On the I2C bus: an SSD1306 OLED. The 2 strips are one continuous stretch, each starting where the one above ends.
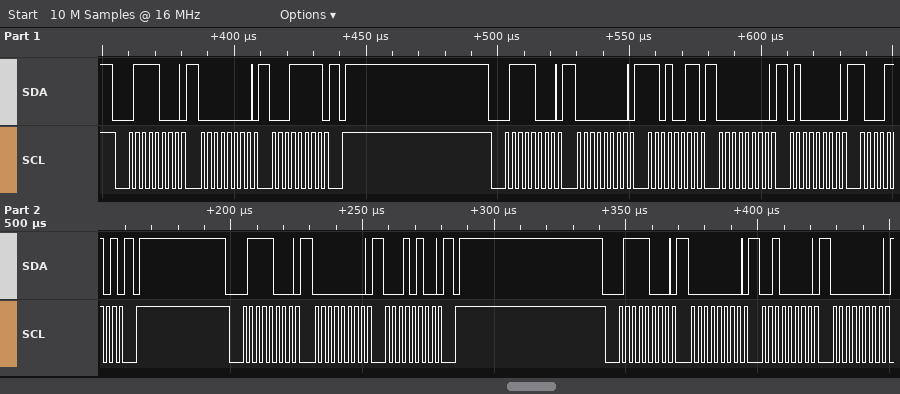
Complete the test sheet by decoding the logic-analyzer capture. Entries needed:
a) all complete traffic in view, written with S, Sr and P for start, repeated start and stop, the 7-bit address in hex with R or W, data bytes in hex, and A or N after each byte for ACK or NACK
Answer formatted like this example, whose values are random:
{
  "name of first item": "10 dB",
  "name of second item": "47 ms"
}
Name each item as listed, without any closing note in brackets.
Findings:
{
  "all complete traffic in view, written with S, Sr and P for start, repeated start and stop, the 7-bit address in hex with R or W, data bytes in hex, and A or N after each byte for ACK or NACK": "S 3CW A 00 A 1F A P S 3CW A 00 A D3 A 00 A 40 A 8D A P S 3CW A 00 A 14 A P S 3CW A 00 A 20 A 00 A"
}
